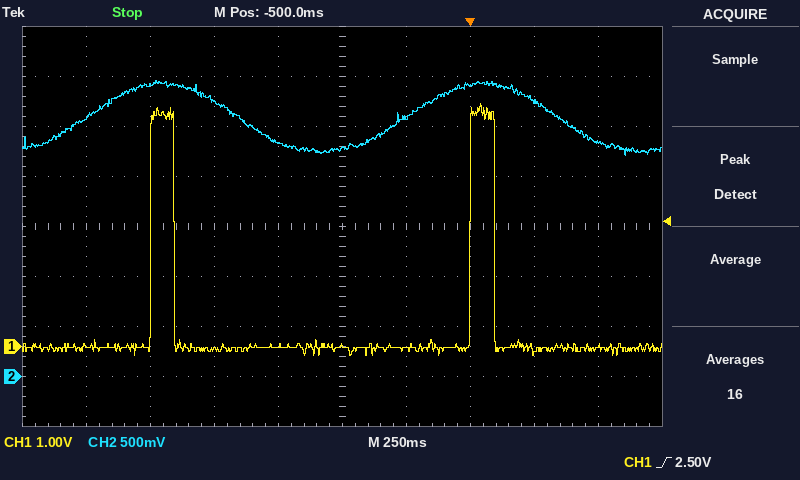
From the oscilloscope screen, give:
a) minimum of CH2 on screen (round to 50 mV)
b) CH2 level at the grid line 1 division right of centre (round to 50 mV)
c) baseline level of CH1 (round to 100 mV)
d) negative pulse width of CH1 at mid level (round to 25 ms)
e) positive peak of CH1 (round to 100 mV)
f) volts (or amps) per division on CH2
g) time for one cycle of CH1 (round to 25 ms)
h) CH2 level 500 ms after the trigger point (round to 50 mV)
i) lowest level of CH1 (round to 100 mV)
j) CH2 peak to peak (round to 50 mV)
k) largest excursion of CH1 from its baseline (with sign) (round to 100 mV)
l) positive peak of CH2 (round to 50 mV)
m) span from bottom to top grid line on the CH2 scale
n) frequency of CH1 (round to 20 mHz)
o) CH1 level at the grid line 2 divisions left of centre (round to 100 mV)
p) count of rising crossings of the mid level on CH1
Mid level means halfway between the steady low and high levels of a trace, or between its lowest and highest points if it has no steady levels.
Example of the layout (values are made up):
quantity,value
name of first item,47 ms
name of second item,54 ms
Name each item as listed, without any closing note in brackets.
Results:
quantity,value
minimum of CH2 on screen,2.20 V
CH2 level at the grid line 1 division right of centre,2.60 V
baseline level of CH1,0.0 V
negative pulse width of CH1 at mid level,1.150 s
positive peak of CH1,4.9 V
volts (or amps) per division on CH2,500 mV
time for one cycle of CH1,1.250 s
CH2 level 500 ms after the trigger point,2.35 V
lowest level of CH1,-200 mV
CH2 peak to peak,750 mV
largest excursion of CH1 from its baseline (with sign),+4.9 V
positive peak of CH2,2.95 V
span from bottom to top grid line on the CH2 scale,4 V
frequency of CH1,800 mHz
CH1 level at the grid line 2 divisions left of centre,-100 mV
count of rising crossings of the mid level on CH1,2
